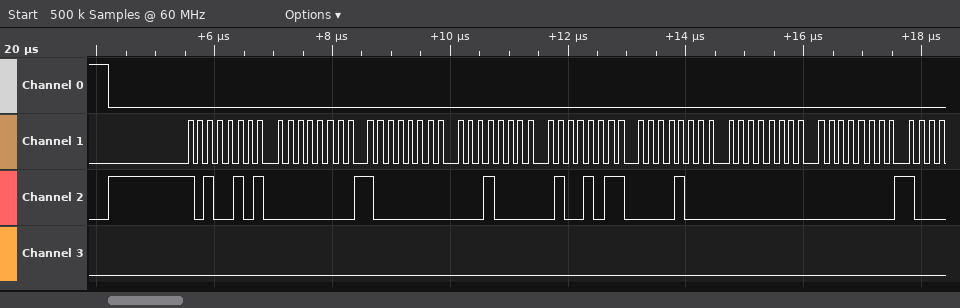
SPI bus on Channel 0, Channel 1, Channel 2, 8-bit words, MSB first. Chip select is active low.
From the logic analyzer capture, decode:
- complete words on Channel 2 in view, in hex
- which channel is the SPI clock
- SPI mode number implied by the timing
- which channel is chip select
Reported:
A5, 00, 80, 10, 4B, 08, 00, 00
Channel 1
0
Channel 0
